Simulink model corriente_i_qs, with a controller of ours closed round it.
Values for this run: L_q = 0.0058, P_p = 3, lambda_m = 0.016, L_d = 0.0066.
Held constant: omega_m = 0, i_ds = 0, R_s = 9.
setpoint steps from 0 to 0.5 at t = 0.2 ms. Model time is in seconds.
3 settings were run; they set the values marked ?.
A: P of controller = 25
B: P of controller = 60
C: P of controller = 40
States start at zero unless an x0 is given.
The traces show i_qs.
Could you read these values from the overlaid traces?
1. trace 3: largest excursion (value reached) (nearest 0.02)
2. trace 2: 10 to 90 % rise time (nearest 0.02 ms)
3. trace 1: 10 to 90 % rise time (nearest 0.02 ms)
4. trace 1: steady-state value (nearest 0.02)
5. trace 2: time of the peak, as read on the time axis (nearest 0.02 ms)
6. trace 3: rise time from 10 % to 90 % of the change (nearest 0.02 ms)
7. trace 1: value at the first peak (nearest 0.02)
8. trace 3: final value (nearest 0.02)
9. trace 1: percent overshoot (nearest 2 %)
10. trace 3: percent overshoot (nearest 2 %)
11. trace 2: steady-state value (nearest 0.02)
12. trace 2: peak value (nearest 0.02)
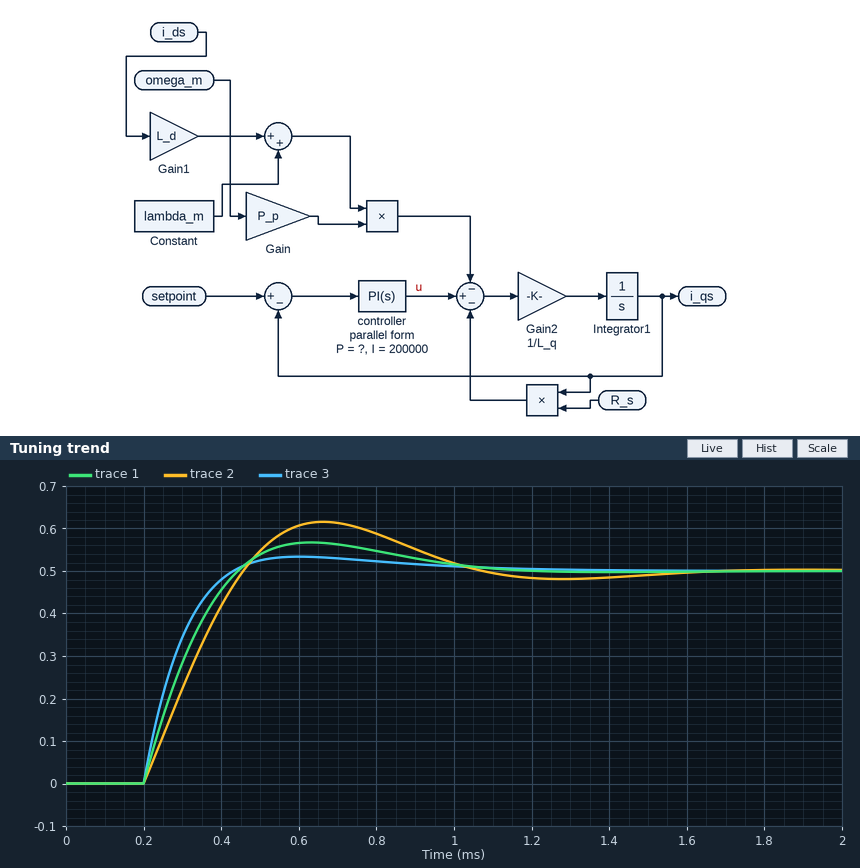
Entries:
0.54
0.20 ms
0.18 ms
0.50
0.66 ms
0.16 ms
0.56
0.50
14 %
6 %
0.50
0.62
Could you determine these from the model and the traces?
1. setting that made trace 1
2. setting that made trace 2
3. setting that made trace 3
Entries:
C
A
B
